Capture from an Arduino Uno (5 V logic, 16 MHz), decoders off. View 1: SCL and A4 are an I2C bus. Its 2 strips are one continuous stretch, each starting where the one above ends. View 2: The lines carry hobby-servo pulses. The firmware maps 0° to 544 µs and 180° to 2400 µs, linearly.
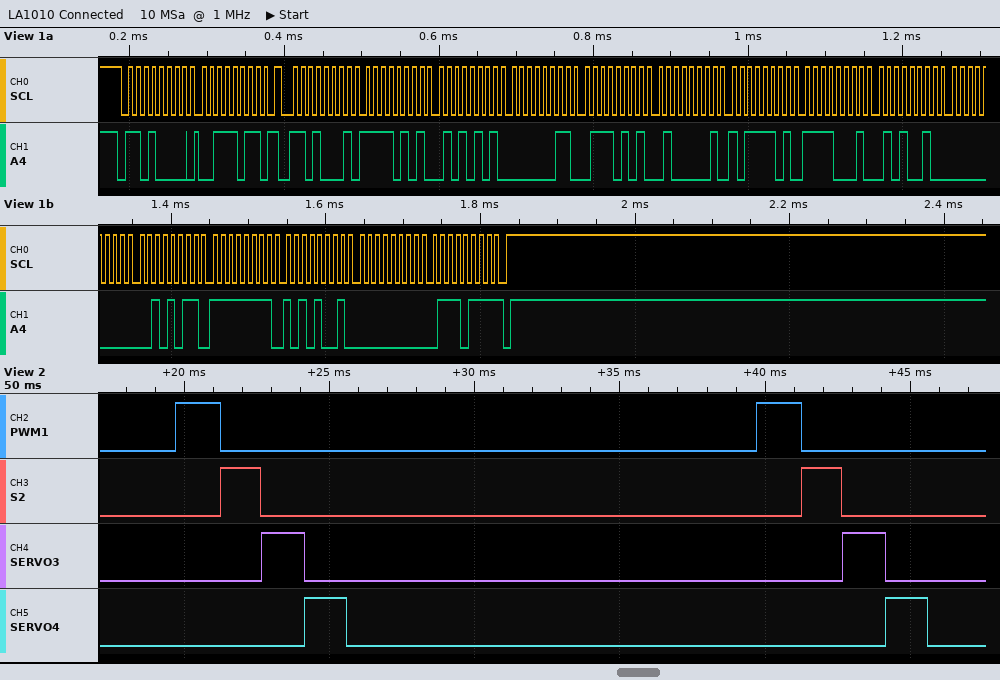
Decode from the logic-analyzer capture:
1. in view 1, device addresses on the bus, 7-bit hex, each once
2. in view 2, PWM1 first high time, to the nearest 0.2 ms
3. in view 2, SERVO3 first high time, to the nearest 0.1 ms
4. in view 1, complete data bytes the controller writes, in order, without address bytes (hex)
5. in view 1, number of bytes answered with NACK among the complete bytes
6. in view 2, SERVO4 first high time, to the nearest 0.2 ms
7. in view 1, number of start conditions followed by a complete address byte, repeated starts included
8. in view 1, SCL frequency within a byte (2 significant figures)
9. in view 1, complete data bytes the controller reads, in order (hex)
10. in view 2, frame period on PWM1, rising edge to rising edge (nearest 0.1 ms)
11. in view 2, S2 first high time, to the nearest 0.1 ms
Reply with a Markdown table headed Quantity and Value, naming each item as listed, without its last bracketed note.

| Quantity | Value |
|---|---|
| in view 1, device addresses on the bus, 7-bit hex, each once | 0x68 |
| in view 2, PWM1 first high time, to the nearest 0.2 ms | 1.6 ms |
| in view 2, SERVO3 first high time, to the nearest 0.1 ms | 1.5 ms |
| in view 1, complete data bytes the controller writes, in order, without address bytes | 3B |
| in view 1, number of bytes answered with NACK among the complete bytes | 1 |
| in view 2, SERVO4 first high time, to the nearest 0.2 ms | 1.4 ms |
| in view 1, number of start conditions followed by a complete address byte, repeated starts included | 2 |
| in view 1, SCL frequency within a byte | 100 kHz |
| in view 1, complete data bytes the controller reads, in order | F5 55 03 75 41 BD F1 52 00 2B FF A9 00 77 |
| in view 2, frame period on PWM1, rising edge to rising edge | 20.0 ms |
| in view 2, S2 first high time, to the nearest 0.1 ms | 1.4 ms |
